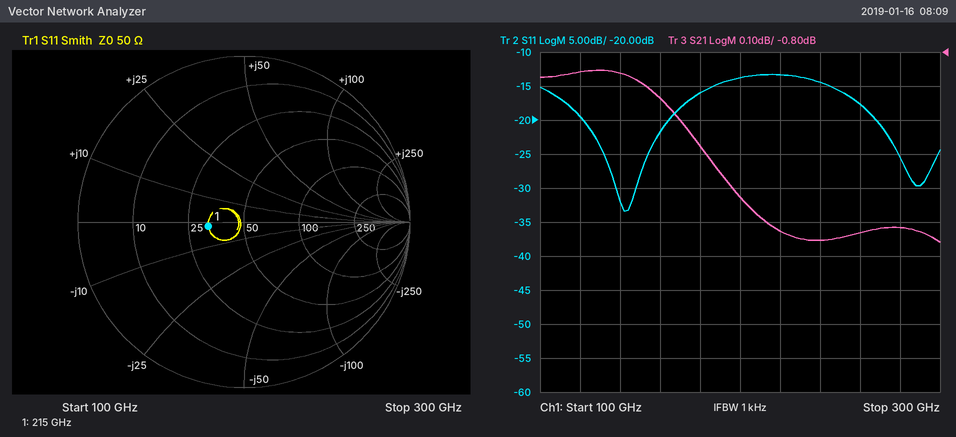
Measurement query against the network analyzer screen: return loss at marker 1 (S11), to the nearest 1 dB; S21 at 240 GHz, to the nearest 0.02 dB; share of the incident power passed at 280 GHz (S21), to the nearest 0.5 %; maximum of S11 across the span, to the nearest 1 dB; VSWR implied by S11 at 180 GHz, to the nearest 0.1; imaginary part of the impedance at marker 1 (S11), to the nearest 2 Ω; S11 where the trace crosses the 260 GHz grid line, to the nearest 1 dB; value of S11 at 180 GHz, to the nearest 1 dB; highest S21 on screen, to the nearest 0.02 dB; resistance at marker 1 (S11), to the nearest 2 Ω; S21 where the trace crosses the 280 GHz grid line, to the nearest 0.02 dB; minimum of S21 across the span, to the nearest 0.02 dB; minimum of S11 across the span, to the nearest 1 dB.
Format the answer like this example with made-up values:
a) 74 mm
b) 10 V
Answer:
a) 13 dB
b) -1.36 dB
c) 74.0 %
d) -13 dB
e) 1.4
f) -2 Ω
g) -18 dB
h) -16 dB
i) -0.86 dB
j) 32 Ω
k) -1.32 dB
l) -1.36 dB
m) -33 dB
